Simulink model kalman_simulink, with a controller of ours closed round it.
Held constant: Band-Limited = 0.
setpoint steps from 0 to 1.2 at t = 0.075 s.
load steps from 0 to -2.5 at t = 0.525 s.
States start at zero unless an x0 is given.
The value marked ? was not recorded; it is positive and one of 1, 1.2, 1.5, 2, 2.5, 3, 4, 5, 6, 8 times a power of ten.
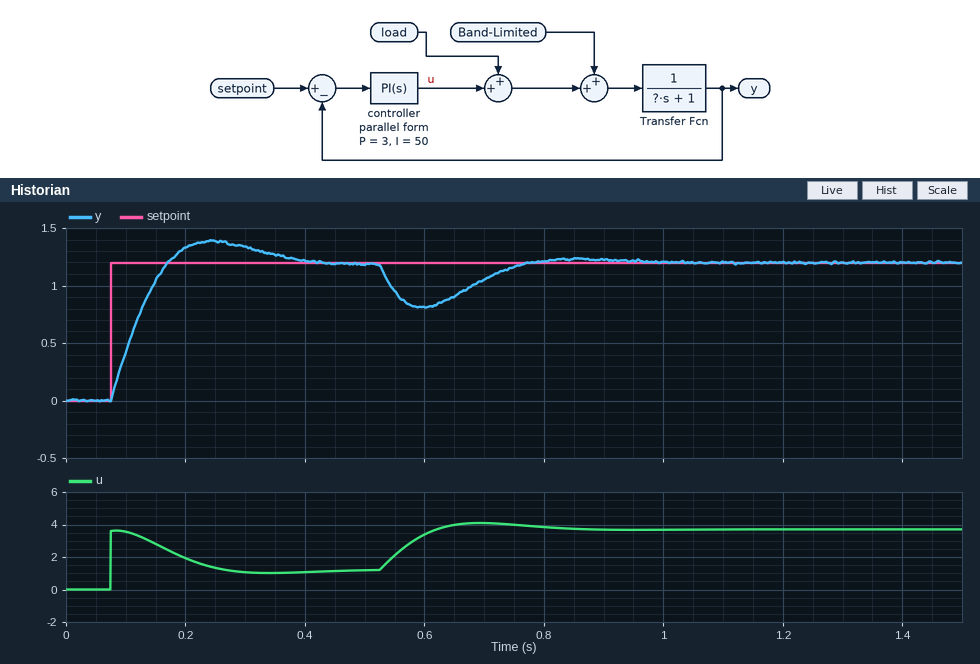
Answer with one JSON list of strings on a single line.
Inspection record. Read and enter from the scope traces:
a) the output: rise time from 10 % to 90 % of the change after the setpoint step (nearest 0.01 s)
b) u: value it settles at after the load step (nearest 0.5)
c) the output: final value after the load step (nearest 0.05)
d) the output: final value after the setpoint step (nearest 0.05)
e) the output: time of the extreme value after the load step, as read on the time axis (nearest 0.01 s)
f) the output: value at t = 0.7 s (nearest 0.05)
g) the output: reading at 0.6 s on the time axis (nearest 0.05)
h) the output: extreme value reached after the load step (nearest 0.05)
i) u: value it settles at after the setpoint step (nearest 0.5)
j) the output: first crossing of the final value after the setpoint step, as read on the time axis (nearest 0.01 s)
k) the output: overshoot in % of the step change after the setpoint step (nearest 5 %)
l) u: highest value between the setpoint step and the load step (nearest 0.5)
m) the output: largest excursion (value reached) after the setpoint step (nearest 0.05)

["0.07 s", "3.5", "1.20", "1.20", "0.60 s", "1.05", "0.80", "0.80", "1.0", "0.17 s", "15 %", "3.5", "1.40"]
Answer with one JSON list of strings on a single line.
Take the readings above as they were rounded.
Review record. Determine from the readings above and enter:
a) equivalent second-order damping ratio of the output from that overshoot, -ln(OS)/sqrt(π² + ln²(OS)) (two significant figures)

["0.52"]
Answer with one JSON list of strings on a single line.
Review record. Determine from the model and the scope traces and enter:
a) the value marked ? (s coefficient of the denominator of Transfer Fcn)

["0.2"]
